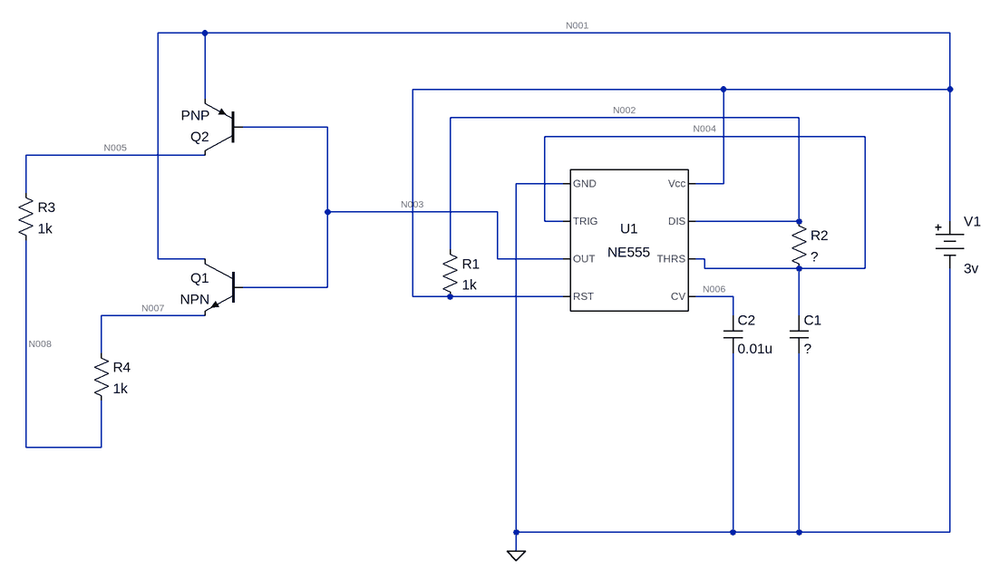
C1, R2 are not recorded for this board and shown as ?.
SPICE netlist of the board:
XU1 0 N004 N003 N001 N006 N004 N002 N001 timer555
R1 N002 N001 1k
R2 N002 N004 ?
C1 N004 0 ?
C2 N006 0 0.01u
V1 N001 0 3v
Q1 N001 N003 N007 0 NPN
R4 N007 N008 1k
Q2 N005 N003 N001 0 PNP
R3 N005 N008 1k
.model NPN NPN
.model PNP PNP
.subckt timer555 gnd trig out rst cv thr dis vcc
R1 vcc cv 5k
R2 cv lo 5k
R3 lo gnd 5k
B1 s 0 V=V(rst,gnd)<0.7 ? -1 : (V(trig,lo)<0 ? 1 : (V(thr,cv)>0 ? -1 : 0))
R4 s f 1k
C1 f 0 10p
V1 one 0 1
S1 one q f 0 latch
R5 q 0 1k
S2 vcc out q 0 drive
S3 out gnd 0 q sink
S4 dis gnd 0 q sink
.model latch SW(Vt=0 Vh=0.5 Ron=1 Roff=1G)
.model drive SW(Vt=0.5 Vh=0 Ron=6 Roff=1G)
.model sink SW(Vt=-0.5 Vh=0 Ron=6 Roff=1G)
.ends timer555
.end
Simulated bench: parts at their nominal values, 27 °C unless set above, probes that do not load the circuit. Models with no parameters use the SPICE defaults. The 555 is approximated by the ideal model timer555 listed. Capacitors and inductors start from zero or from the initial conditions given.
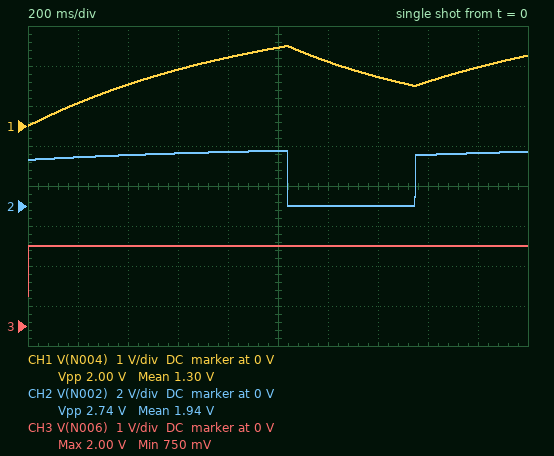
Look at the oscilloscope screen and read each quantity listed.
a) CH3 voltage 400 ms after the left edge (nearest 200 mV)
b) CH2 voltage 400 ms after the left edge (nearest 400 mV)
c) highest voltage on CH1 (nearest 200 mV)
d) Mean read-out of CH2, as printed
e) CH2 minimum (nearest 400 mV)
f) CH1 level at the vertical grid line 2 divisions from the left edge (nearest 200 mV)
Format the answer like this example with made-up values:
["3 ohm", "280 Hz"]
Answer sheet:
["2.0 V", "2.4 V", "2.0 V", "1.94 V", "0 V", "1.0 V"]
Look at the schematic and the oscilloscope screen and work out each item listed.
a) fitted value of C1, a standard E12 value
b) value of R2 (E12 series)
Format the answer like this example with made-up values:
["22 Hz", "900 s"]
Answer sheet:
["220 µF", "3.3 kΩ"]
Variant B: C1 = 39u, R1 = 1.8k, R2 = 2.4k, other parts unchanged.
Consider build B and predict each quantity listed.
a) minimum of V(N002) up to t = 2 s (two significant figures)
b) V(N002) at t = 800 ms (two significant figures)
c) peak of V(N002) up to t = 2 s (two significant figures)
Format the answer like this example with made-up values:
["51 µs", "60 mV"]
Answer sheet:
["12 mV", "2.2 V", "2.6 V"]
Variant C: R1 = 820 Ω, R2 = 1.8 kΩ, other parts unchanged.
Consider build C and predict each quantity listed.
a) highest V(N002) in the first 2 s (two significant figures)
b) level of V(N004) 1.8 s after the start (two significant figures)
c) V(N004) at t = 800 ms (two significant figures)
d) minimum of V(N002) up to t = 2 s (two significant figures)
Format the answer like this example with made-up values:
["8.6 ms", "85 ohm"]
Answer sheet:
["2.7 V", "1.6 V", "1.3 V", "25 mV"]
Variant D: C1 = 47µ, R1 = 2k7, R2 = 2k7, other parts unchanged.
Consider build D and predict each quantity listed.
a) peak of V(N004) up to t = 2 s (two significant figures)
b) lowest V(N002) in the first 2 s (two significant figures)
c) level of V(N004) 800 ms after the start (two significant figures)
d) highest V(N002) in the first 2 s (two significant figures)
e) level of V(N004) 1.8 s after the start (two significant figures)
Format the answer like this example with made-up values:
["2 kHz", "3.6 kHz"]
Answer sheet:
["2.0 V", "8.9 mV", "2.0 V", "2.5 V", "1.7 V"]
